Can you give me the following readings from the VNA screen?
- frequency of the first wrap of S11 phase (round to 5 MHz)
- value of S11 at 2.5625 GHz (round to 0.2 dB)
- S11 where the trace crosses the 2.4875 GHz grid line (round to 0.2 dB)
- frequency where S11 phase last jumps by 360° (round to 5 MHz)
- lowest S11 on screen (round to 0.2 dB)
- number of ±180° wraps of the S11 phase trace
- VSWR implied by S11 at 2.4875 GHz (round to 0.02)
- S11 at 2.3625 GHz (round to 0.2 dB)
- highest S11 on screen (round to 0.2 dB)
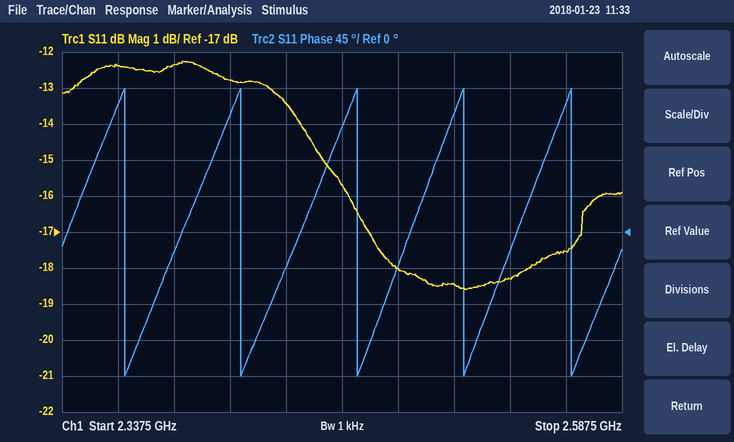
2.365 GHz
-17.6 dB
-18.0 dB
2.565 GHz
-18.6 dB
5
1.28
-12.4 dB
-12.2 dB
